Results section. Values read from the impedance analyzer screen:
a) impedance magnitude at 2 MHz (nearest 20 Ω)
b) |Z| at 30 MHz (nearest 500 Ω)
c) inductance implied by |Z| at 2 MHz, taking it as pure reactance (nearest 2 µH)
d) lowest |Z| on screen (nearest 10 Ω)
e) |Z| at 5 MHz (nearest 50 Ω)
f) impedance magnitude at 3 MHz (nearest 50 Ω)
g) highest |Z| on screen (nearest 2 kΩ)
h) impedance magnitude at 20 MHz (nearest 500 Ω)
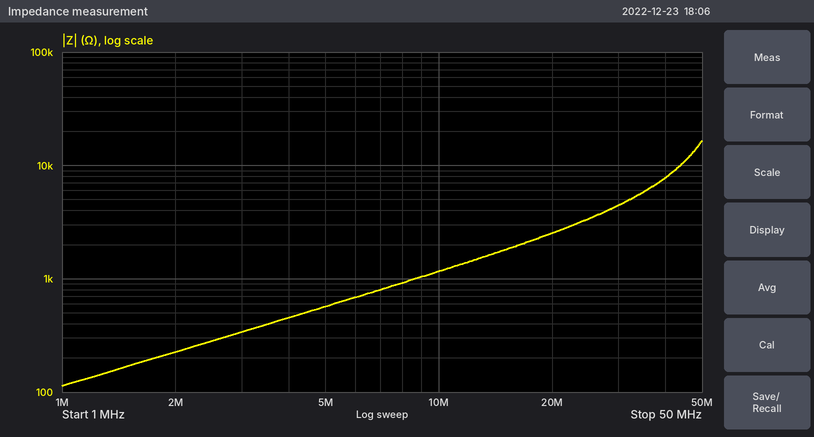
220 Ω
4.5 kΩ
18 µH
110 Ω
550 Ω
350 Ω
16 kΩ
2.5 kΩ
